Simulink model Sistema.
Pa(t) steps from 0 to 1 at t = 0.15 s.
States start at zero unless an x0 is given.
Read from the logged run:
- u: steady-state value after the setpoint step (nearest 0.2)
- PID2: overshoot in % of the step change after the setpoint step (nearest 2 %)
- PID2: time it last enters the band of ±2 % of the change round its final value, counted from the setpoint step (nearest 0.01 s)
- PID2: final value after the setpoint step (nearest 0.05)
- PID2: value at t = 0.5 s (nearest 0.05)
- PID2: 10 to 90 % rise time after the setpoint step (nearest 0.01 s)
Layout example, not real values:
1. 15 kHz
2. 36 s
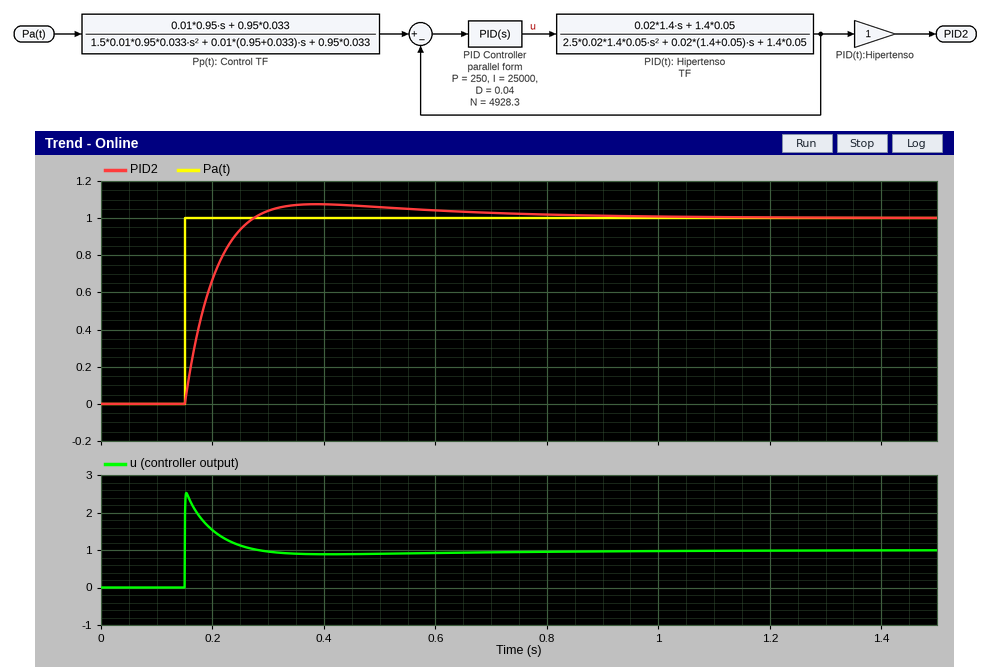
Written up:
1. 1.0
2. 8 %
3. 0.64 s
4. 1.00
5. 1.05
6. 0.08 s
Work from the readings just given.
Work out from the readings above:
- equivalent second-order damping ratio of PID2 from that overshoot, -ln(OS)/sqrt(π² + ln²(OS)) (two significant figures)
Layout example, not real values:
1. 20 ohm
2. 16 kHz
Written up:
1. 0.63
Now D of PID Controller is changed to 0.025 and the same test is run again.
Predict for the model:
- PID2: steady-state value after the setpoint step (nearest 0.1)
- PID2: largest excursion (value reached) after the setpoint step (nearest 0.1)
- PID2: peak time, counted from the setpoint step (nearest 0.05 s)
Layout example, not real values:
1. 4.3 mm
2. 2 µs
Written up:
1. 1.0
2. 1.1
3. 0.25 s
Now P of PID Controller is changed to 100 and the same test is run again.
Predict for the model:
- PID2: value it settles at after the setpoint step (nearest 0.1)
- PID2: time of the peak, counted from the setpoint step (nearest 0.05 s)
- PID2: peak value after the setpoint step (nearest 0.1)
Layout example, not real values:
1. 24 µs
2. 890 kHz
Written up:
1. 1.0
2. 0.25 s
3. 1.1
